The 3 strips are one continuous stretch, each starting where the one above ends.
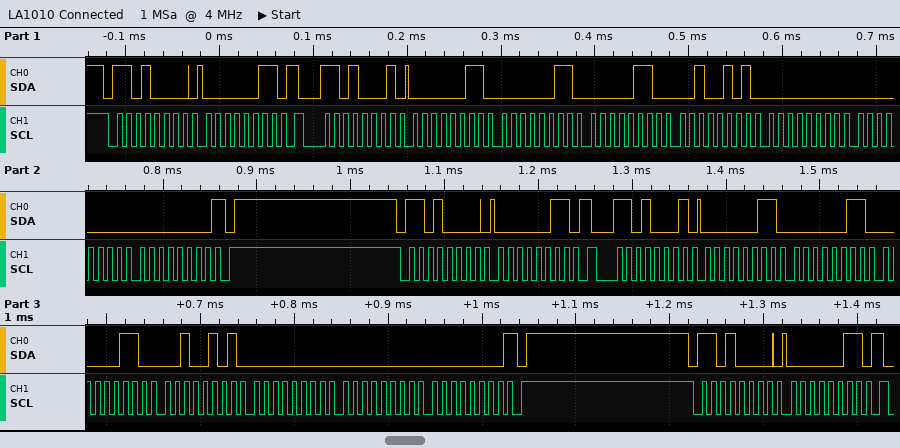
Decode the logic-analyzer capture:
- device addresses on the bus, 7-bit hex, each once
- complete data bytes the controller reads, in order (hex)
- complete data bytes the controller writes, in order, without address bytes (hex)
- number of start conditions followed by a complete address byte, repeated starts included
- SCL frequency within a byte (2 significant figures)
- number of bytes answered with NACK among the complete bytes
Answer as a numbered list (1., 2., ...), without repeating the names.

1. 0x68
2. 03 03 06 25 00 00 00 03 03 06 25 00 00 00
3. 03 03 03
4. 5
5. 100 kHz
6. 2
